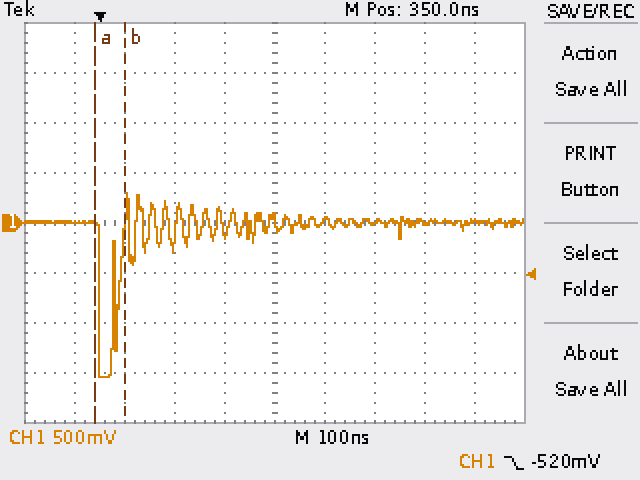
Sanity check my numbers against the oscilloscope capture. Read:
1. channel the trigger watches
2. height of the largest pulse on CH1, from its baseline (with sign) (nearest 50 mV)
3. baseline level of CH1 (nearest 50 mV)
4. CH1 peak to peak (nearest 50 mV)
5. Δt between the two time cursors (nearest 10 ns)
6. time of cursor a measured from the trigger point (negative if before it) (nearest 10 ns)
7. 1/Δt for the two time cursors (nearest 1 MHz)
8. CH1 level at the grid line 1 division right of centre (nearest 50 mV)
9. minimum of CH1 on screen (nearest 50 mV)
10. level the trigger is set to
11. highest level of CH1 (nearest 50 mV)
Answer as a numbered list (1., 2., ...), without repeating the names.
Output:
1. CH1
2. -1.55 V
3. 0 mV
4. 1.85 V
5. 60 ns
6. -10 ns
7. 17 MHz
8. 0 mV
9. -1.55 V
10. -520 mV
11. 300 mV
